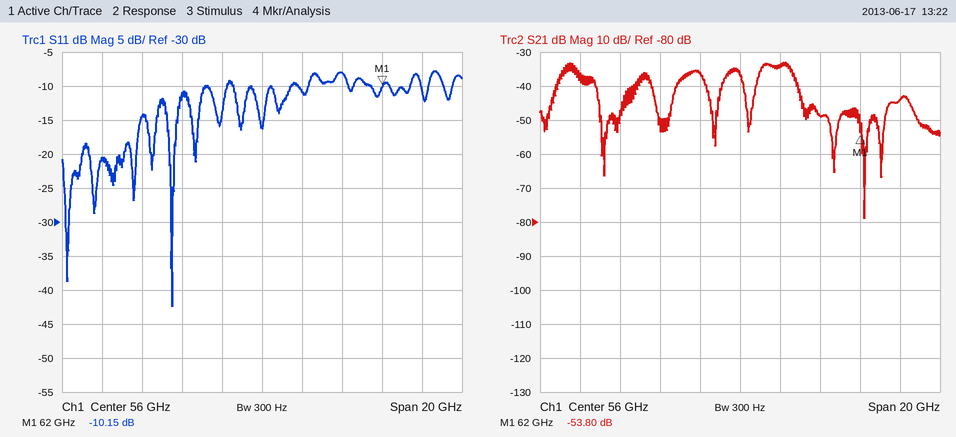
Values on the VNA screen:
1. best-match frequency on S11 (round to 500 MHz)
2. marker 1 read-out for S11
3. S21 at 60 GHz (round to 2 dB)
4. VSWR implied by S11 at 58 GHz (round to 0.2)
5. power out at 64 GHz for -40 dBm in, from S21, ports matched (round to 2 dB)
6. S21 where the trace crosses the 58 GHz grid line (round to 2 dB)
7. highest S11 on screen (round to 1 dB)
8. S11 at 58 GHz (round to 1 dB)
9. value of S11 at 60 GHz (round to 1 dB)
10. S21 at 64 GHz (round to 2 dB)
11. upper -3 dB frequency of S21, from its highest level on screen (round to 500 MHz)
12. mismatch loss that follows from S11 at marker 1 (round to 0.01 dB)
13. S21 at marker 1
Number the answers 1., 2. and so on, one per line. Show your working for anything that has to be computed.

1. 51.5 GHz
2. -10.15 dB
3. -48 dB
4. |Γ| = 10^(-11/20) = 0.2818; VSWR = (1 + 0.2818)/(1 − 0.2818) ≈ 1.8
5. -40 dBm + (-44 dB) = -84 dBm
6. -34 dB
7. -8 dB
8. -11 dB
9. -8 dB
10. -44 dB
11. 58.5 GHz
12. −10 log10(1 − 10^(-10.15/10)) ≈ 0.44 dB
13. -53.80 dB
